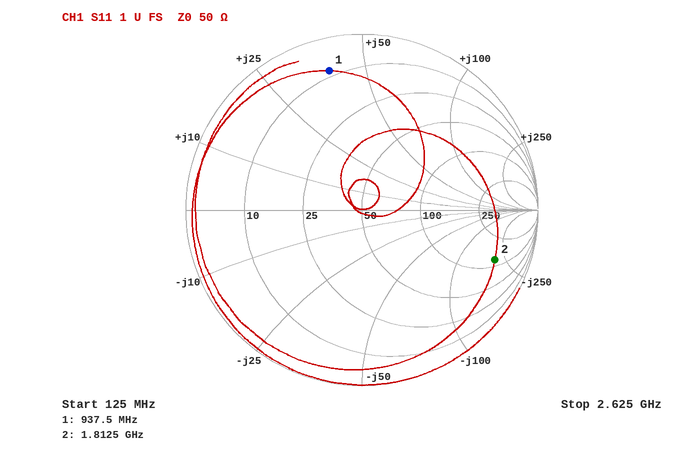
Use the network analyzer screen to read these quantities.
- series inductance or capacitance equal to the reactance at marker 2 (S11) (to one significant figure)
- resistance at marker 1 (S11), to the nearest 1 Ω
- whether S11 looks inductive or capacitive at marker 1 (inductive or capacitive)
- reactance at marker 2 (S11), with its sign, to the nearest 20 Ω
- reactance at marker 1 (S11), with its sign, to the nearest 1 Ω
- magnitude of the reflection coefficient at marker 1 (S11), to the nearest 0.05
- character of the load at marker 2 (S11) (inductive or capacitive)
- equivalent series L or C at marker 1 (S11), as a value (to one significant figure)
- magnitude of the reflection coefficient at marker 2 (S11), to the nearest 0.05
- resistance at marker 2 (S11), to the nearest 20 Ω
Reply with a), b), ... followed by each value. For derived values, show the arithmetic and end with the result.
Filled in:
a) C = 1/(2π × 1.8125 GHz × 200 Ω) ≈ 439 fF, so 400 fF to one significant figure
b) 8 Ω
c) inductive
d) -200 Ω
e) +39 Ω
f) 0.80
g) capacitive
h) L = 39 Ω/(2π × 937.5 MHz) ≈ 7 nH
i) 0.80
j) 120 Ω
